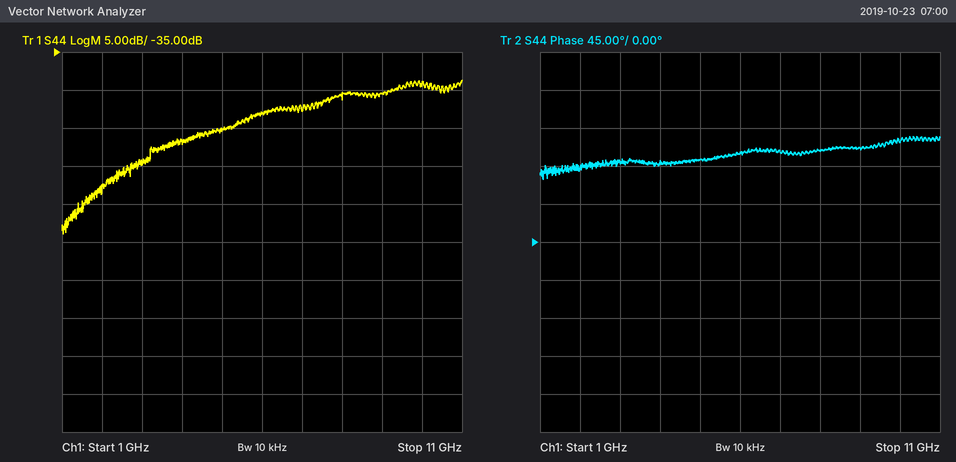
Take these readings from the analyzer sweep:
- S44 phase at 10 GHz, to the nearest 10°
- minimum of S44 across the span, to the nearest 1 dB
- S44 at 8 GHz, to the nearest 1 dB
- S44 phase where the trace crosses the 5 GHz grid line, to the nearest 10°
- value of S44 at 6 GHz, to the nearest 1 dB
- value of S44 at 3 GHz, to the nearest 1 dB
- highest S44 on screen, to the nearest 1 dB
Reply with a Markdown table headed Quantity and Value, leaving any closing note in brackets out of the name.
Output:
| Quantity | Value |
|---|---|
| S44 phase at 10 GHz, to the nearest 10° | 120° |
| minimum of S44 across the span, to the nearest 1 dB | -59 dB |
| S44 at 8 GHz, to the nearest 1 dB | -41 dB |
| S44 phase where the trace crosses the 5 GHz grid line, to the nearest 10° | 100° |
| value of S44 at 6 GHz, to the nearest 1 dB | -43 dB |
| value of S44 at 3 GHz, to the nearest 1 dB | -50 dB |
| highest S44 on screen, to the nearest 1 dB | -39 dB |
